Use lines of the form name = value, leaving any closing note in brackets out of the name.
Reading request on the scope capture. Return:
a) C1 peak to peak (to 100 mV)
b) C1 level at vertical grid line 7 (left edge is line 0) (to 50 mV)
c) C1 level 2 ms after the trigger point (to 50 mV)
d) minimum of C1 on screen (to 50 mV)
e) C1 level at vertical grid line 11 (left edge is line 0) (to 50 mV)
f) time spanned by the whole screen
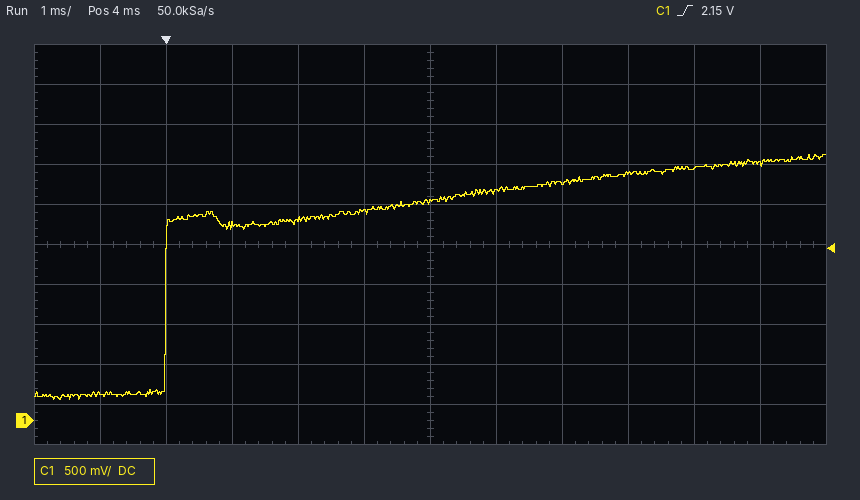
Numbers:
C1 peak to peak = 3.10 V
C1 level at vertical grid line 7 (left edge is line 0) = 2.85 V
C1 level 2 ms after the trigger point = 2.50 V
minimum of C1 on screen = 250 mV
C1 level at vertical grid line 11 (left edge is line 0) = 3.20 V
time spanned by the whole screen = 12 ms
